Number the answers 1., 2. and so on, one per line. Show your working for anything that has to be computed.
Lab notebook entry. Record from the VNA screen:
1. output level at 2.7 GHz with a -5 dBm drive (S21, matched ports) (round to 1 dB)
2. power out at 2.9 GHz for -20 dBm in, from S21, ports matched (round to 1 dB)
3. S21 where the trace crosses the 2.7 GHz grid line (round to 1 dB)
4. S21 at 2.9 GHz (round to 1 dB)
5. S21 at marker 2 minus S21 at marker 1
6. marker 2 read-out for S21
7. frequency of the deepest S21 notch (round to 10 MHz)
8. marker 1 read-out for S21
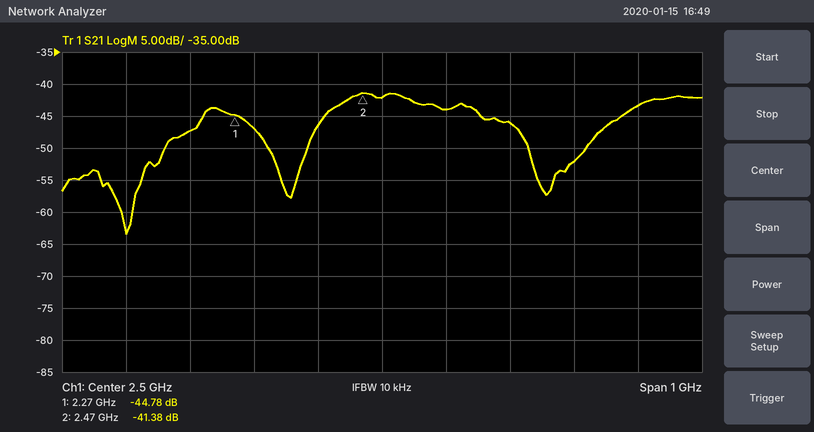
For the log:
1. -5 dBm + (-46 dB) = -51 dBm
2. -20 dBm + (-43 dB) = -63 dBm
3. -46 dB
4. -43 dB
5. -41.38 − (-44.78) = 3.40 dB
6. -41.38 dB
7. 2.10 GHz
8. -44.78 dB
